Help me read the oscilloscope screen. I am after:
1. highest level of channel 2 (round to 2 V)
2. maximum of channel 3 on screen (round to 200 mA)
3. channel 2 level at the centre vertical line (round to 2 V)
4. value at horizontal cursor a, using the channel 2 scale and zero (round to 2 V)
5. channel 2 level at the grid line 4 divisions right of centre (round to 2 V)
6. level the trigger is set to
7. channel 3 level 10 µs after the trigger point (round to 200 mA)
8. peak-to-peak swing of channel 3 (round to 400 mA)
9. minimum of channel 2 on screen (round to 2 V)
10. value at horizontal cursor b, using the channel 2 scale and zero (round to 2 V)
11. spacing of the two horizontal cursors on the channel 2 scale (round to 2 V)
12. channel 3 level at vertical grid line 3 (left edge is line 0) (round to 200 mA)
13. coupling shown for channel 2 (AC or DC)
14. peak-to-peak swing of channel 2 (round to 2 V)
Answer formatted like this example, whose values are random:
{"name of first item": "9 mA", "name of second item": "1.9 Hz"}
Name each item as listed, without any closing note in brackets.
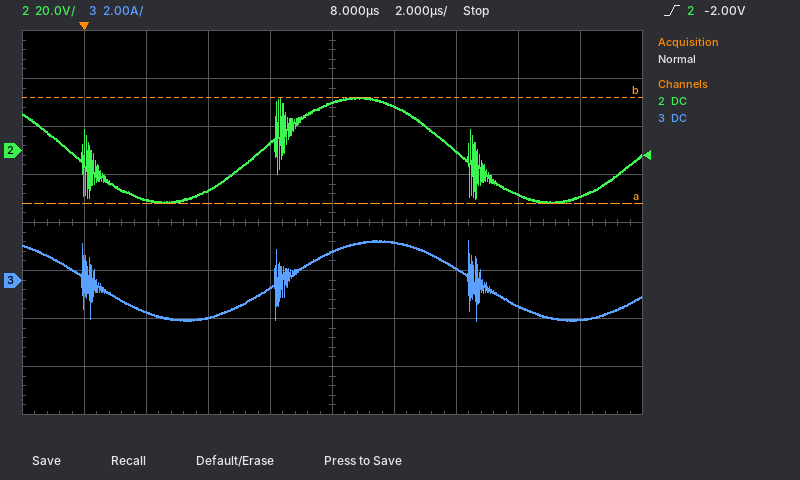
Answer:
{"highest level of channel 2": "22 V", "maximum of channel 3 on screen": "1.6 A", "channel 2 level at the centre vertical line": "20 V", "value at horizontal cursor a, using the channel 2 scale and zero": "-22 V", "channel 2 level at the grid line 4 divisions right of centre": "-20 V", "level the trigger is set to": "-2.00 V", "channel 3 level 10 µs after the trigger point": "1.6 A", "peak-to-peak swing of channel 3": "3.2 A", "minimum of channel 2 on screen": "-22 V", "value at horizontal cursor b, using the channel 2 scale and zero": "22 V", "spacing of the two horizontal cursors on the channel 2 scale": "44 V", "channel 3 level at vertical grid line 3 (left edge is line 0)": "-1.6 A", "coupling shown for channel 2": "DC", "peak-to-peak swing of channel 2": "44 V"}
